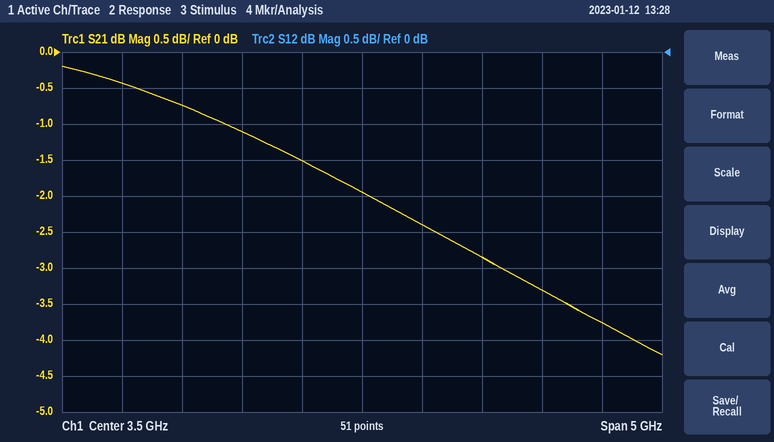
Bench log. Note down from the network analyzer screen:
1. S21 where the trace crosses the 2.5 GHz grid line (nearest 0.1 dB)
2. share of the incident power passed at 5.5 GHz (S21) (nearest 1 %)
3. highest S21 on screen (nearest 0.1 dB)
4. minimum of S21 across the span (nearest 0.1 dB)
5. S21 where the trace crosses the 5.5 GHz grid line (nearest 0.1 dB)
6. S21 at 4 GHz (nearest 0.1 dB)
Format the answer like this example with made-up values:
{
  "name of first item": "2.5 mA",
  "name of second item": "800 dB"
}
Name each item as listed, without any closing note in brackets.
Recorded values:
{
  "S21 where the trace crosses the 2.5 GHz grid line": "-1.1 dB",
  "share of the incident power passed at 5.5 GHz (S21)": "42 %",
  "highest S21 on screen": "-0.2 dB",
  "minimum of S21 across the span": "-4.2 dB",
  "S21 where the trace crosses the 5.5 GHz grid line": "-3.8 dB",
  "S21 at 4 GHz": "-2.4 dB"
}
